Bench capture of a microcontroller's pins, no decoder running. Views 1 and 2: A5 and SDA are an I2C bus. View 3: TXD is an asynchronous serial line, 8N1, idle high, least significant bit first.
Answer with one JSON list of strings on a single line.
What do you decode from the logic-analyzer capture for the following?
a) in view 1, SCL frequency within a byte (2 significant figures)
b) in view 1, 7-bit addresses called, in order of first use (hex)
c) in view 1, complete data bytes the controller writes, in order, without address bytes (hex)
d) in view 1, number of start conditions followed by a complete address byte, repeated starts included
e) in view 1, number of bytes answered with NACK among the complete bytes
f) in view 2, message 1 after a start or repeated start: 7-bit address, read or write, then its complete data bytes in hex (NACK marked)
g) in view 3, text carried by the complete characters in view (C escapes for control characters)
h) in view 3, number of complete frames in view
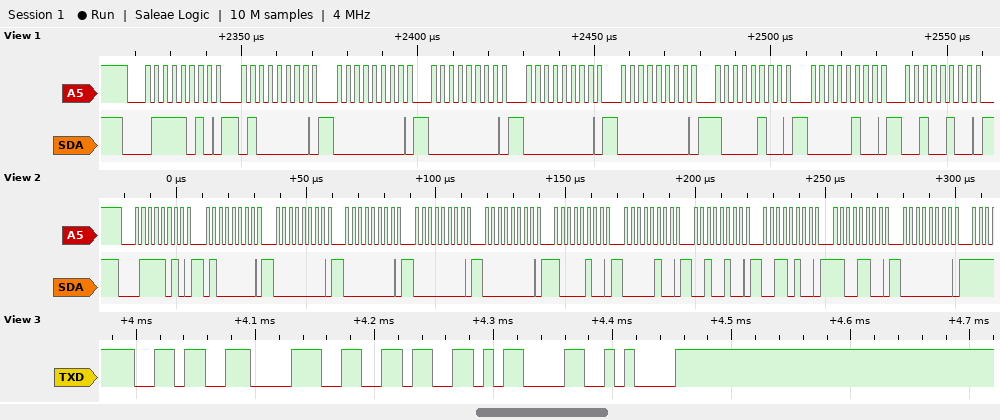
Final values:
["400 kHz", "0x3D", "40 00 00 00 00 84 04 24", "1", "0", "0x3D write: 40 00 00 00 00 84 04 24 34 CC 00", "\"686\\r\\n\"", "5"]
